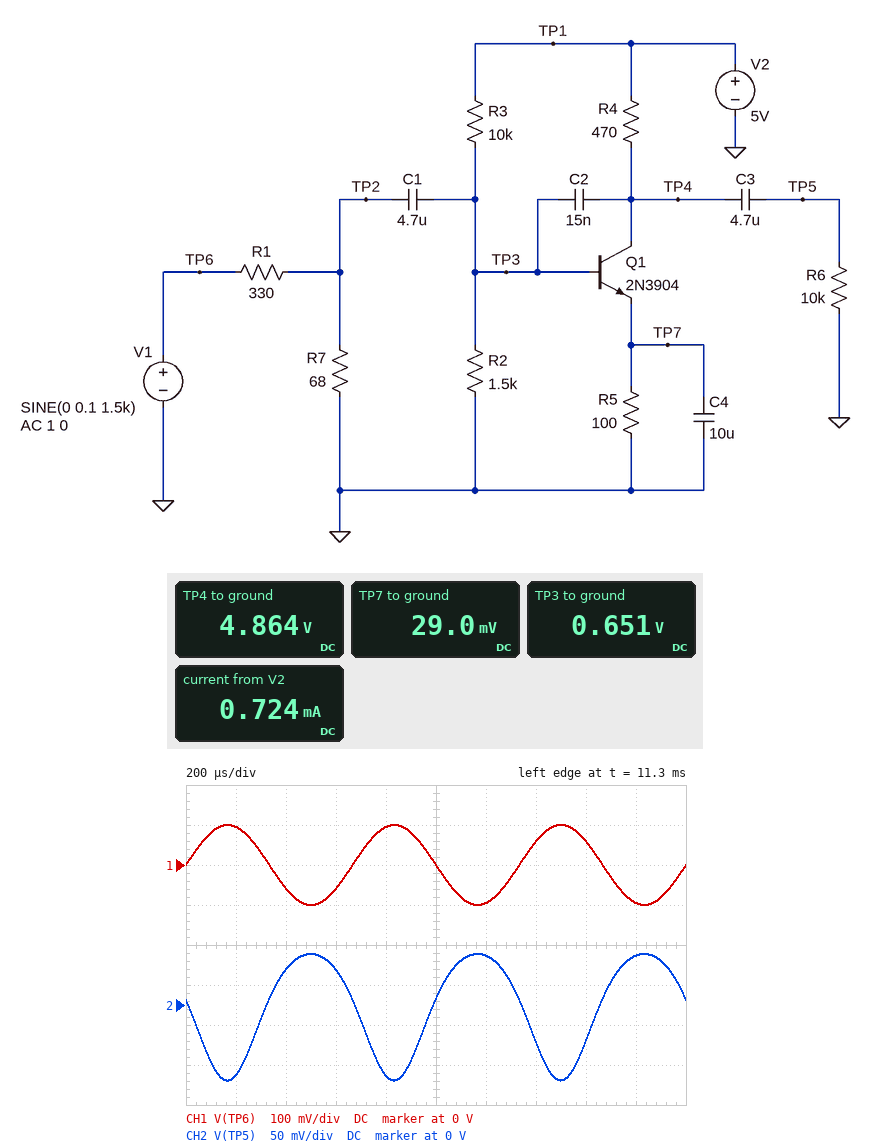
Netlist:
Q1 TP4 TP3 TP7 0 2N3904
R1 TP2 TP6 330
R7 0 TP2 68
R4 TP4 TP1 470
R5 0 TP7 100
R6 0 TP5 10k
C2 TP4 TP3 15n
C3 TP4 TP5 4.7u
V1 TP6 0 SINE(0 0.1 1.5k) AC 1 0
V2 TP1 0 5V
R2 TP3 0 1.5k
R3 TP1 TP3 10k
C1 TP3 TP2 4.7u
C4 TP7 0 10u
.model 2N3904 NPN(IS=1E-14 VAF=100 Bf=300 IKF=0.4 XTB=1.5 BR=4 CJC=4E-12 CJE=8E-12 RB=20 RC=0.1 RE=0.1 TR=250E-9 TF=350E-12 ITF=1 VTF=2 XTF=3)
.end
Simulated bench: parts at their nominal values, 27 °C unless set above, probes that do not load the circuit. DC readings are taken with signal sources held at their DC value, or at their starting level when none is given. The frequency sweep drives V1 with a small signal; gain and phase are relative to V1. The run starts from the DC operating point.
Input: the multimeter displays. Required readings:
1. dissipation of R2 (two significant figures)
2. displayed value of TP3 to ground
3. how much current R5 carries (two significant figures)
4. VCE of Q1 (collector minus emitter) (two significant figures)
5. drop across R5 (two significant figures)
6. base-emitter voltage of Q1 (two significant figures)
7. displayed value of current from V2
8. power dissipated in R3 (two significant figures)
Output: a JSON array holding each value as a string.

["280 µW", "0.651 V", "290 µA", "4.8 V", "29 mV", "620 mV", "0.724 mA", "1.9 mW"]
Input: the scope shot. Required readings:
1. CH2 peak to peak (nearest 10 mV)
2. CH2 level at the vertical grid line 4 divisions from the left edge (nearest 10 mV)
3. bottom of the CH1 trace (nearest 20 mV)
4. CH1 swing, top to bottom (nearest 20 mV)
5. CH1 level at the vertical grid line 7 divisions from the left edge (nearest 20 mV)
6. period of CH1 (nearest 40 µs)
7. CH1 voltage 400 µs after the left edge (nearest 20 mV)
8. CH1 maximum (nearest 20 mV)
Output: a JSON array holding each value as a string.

["160 mV", "-90 mV", "-100 mV", "200 mV", "60 mV", "680 µs", "-60 mV", "100 mV"]
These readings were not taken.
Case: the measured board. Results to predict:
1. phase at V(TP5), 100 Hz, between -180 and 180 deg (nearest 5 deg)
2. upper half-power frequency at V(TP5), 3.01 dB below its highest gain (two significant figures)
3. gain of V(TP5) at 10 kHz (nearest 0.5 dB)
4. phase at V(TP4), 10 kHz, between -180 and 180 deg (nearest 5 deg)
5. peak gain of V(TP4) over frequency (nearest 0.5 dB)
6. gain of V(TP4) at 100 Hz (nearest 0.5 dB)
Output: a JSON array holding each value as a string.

["-150 deg", "15 kHz", "-3.5 dB", "140 deg", "-2.0 dB", "-7.5 dB"]
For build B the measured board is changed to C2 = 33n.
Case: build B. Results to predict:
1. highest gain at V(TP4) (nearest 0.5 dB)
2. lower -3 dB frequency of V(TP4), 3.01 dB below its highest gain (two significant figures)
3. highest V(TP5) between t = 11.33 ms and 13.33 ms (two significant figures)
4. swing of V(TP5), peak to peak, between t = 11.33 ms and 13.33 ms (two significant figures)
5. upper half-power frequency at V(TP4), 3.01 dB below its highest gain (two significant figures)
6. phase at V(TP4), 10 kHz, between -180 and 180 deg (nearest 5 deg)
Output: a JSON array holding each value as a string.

["-2.5 dB", "220 Hz", "62 mV", "150 mV", "7.1 kHz", "115 deg"]
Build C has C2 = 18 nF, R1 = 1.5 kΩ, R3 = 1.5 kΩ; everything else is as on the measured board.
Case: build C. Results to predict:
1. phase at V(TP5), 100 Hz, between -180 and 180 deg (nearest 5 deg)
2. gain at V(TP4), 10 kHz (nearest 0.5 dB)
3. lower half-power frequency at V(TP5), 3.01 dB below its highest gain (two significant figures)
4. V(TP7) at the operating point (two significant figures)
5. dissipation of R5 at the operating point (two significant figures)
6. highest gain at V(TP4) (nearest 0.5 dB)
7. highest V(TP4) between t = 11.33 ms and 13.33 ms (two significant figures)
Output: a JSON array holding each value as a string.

["40 deg", "-43.5 dB", "100 Hz", "960 mV", "9.2 mW", "-41.5 dB", "990 mV"]
